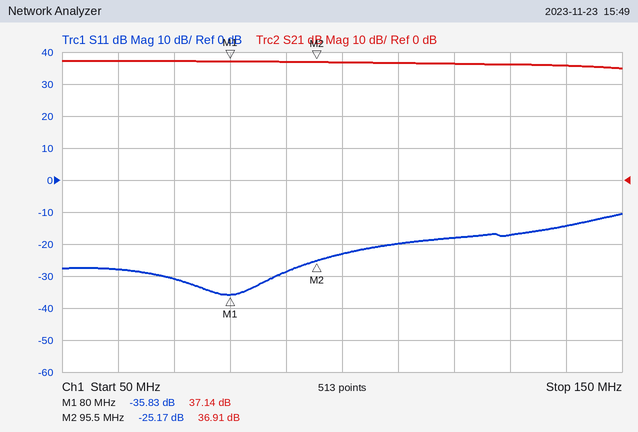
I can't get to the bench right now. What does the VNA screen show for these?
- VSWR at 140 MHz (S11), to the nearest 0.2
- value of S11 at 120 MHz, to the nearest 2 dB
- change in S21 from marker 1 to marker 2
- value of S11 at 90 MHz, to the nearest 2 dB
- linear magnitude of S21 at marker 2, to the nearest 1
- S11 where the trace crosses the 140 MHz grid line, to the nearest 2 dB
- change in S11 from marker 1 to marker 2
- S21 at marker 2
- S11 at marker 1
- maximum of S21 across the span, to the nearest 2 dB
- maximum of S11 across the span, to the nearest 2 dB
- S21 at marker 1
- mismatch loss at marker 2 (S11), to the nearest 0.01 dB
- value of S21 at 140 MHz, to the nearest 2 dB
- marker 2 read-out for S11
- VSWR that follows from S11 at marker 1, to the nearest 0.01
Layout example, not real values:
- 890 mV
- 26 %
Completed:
- 1.4
- -18 dB
- -0.23 dB
- -28 dB
- 70
- -14 dB
- 10.66 dB
- 36.91 dB
- -35.83 dB
- 38 dB
- -10 dB
- 37.14 dB
- 0.01 dB
- 36 dB
- -25.17 dB
- 1.03
